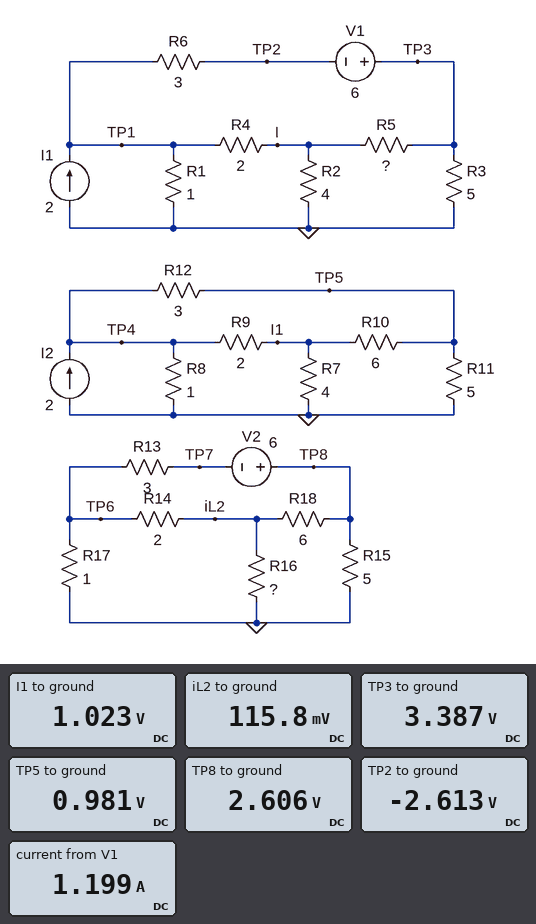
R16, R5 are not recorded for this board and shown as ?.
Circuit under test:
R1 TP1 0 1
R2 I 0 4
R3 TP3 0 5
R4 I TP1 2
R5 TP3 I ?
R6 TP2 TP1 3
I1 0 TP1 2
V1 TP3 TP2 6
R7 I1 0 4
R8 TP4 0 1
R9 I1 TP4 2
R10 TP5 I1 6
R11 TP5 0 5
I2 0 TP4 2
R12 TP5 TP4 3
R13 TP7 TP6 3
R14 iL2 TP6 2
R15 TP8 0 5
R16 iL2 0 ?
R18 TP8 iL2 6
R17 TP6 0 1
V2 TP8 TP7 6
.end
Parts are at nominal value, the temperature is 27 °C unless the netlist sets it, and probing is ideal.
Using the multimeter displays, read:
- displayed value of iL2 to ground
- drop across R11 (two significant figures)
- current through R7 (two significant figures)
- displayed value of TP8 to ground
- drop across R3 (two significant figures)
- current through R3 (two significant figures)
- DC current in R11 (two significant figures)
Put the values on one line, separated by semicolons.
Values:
115.8 mV; 980 mV; 260 mA; 2.606 V; 3.4 V; 680 mA; 200 mA
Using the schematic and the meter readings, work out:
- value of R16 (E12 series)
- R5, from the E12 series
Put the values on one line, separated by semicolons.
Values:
1.8 Ω; 3.9 Ω
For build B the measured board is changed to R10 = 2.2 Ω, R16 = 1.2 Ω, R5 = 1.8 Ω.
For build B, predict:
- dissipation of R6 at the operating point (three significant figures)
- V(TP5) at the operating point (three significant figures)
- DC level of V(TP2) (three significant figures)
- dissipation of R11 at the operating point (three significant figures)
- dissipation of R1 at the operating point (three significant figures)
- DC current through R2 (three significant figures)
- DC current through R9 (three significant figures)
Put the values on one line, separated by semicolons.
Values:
5.36 W; 990 mV; -3.02 V; 196 mW; 983 mW; 412 mA; 266 mA
